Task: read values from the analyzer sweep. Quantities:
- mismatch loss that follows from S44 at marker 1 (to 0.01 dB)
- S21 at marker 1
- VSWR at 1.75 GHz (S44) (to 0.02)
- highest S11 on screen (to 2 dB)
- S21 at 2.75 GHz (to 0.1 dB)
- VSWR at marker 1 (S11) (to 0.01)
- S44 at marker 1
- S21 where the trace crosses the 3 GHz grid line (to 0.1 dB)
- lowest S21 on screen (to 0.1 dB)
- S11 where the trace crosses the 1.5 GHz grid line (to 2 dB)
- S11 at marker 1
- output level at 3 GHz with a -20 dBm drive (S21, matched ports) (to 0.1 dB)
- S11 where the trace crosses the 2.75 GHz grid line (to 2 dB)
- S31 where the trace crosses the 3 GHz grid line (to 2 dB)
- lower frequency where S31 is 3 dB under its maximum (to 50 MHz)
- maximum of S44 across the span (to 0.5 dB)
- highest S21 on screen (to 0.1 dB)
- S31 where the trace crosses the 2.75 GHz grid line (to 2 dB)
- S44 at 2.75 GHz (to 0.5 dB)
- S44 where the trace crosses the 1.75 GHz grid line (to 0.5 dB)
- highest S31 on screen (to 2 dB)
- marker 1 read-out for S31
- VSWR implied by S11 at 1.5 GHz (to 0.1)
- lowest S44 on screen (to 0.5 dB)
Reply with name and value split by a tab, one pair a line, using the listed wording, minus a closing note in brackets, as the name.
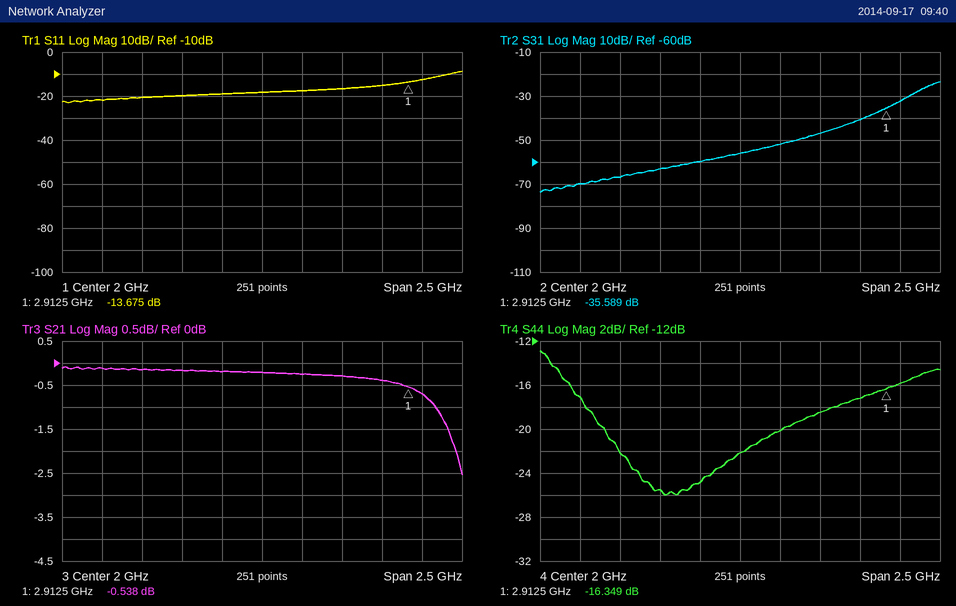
mismatch loss that follows from S44 at marker 1	0.10 dB
S21 at marker 1	-0.538 dB
VSWR at 1.75 GHz (S44)	1.12
highest S11 on screen	-8 dB
S21 at 2.75 GHz	-0.4 dB
VSWR at marker 1 (S11)	1.52
S44 at marker 1	-16.349 dB
S21 where the trace crosses the 3 GHz grid line	-0.7 dB
lowest S21 on screen	-2.5 dB
S11 where the trace crosses the 1.5 GHz grid line	-20 dB
S11 at marker 1	-13.675 dB
output level at 3 GHz with a -20 dBm drive (S21, matched ports)	-20.7 dBm
S11 where the trace crosses the 2.75 GHz grid line	-16 dB
S31 where the trace crosses the 3 GHz grid line	-32 dB
lower frequency where S31 is 3 dB under its maximum	3.15 GHz
maximum of S44 across the span	-13.0 dB
highest S21 on screen	-0.1 dB
S31 where the trace crosses the 2.75 GHz grid line	-40 dB
S44 at 2.75 GHz	-17.0 dB
S44 where the trace crosses the 1.75 GHz grid line	-25.0 dB
highest S31 on screen	-24 dB
marker 1 read-out for S31	-35.589 dB
VSWR implied by S11 at 1.5 GHz	1.2
lowest S44 on screen	-26.0 dB
